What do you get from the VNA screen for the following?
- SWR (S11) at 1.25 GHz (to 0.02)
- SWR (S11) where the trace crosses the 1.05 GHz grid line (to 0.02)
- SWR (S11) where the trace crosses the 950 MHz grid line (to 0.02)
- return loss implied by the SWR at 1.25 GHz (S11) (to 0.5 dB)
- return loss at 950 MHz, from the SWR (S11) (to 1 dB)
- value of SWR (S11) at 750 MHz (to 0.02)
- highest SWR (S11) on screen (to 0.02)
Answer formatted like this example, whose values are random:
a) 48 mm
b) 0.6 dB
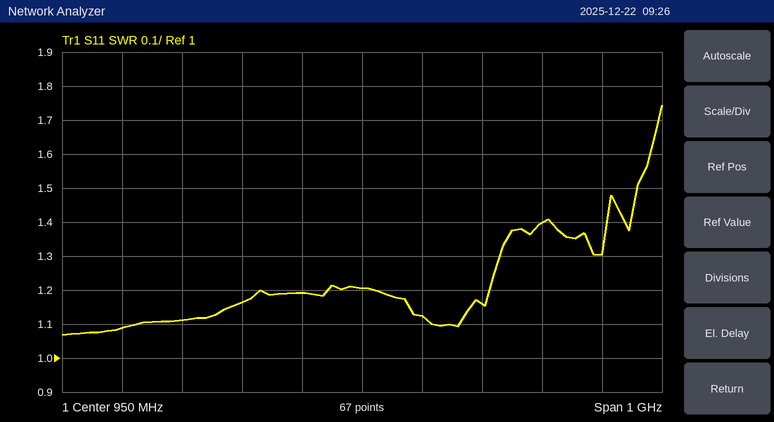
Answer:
a) 1.40
b) 1.12
c) 1.20
d) 15.5 dB
e) 21 dB
f) 1.16
g) 1.74
